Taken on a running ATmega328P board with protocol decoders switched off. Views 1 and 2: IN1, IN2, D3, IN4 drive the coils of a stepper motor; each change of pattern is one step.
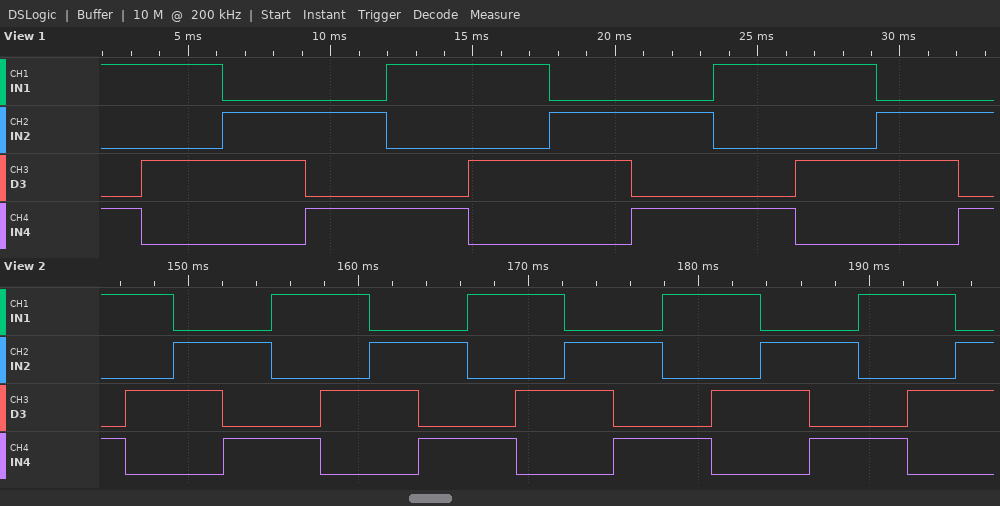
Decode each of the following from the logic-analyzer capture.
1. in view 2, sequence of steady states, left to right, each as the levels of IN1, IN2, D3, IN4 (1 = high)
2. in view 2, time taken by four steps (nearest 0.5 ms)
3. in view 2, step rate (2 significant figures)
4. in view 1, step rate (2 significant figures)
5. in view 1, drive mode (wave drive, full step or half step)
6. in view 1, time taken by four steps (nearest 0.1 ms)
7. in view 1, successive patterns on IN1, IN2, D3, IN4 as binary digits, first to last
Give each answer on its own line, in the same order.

1001 1010 0110 0101 1001 1010 0110 0101 1001 1010 0110 0101 1001 1010 0110 0101 1001 1010 0110
11.5 ms
350 steps/s
350 steps/s
full step
11.5 ms
1001 1010 0110 0101 1001 1010 0110 0101 1001 1010 0110 0101
